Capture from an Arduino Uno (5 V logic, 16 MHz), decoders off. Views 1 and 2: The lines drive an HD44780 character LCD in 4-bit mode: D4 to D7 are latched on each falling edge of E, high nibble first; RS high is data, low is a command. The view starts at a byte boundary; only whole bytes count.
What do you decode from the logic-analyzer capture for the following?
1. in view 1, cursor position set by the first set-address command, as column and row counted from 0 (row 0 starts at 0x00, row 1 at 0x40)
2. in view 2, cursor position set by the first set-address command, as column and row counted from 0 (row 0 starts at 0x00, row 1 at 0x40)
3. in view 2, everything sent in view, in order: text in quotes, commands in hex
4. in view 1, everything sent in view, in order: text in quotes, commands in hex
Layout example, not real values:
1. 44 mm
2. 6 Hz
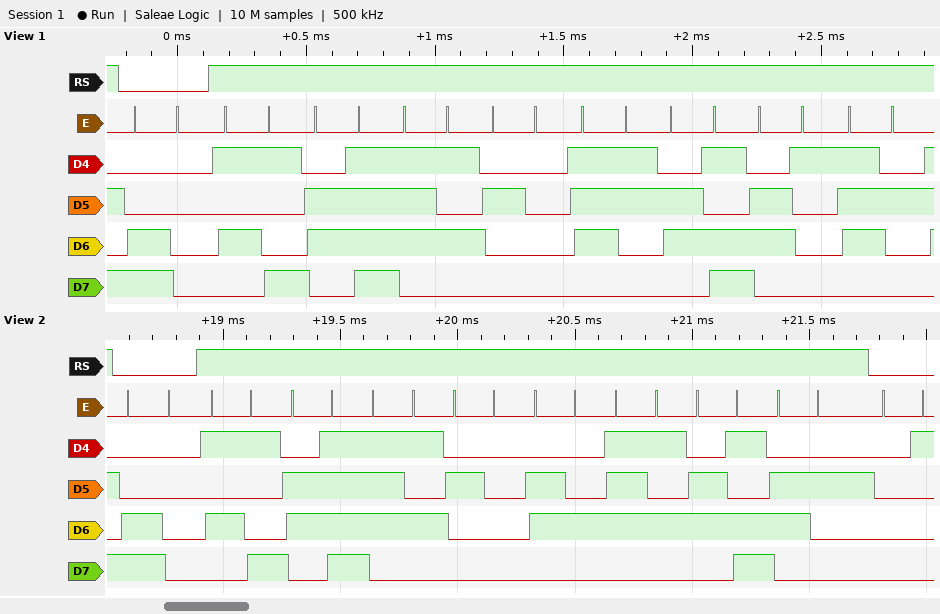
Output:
1. column 0, row 1
2. column 0, row 1
3. 0xC0 "You dumb" 0x01
4. 0xC0 "You smar"
